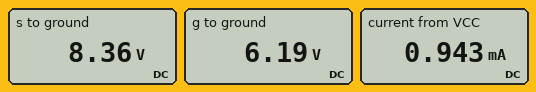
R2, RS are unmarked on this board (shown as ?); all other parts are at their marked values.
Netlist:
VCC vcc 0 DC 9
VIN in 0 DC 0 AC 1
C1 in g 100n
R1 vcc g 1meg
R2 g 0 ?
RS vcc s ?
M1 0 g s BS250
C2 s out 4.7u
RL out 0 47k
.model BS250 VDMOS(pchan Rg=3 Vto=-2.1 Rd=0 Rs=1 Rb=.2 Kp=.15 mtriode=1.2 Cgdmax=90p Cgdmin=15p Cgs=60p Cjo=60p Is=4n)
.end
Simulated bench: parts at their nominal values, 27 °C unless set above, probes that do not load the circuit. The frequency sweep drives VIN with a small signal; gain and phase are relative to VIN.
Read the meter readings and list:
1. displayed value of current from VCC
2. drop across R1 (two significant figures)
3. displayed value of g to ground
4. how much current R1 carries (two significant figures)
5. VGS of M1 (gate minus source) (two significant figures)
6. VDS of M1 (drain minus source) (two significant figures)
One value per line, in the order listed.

0.943 mA
2.8 V
6.19 V
2.8 µA
-2.2 V
-8.4 V
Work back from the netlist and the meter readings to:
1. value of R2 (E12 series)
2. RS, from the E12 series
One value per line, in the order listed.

2.2 MΩ
680 Ω
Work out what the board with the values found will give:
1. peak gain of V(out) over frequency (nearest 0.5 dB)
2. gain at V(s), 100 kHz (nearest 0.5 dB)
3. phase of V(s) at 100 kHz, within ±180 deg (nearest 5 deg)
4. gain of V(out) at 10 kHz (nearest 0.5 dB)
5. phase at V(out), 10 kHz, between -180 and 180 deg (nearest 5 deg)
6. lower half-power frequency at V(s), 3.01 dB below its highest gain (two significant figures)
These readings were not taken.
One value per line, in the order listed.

-1.0 dB
-1.0 dB
0 deg
-1.0 dB
0 deg
2.3 Hz
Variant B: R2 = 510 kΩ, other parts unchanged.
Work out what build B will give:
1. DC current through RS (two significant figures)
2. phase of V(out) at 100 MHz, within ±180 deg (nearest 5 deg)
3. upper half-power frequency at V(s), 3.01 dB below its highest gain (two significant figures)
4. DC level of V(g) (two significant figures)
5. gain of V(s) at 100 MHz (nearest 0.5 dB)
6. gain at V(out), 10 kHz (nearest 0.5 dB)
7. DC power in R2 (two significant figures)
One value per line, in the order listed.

5.3 mA
-10 deg
580 MHz
3.0 V
-1.5 dB
-0.5 dB
18 µW
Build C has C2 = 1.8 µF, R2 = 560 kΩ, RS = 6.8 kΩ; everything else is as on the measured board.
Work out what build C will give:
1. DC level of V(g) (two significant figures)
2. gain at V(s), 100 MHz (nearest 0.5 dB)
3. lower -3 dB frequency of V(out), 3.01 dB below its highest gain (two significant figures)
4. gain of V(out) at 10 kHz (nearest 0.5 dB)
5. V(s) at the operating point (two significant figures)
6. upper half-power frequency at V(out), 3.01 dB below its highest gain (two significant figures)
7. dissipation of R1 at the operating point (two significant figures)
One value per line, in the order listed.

3.2 V
-2.5 dB
5.1 Hz
0 dB
5.4 V
460 MHz
33 µW
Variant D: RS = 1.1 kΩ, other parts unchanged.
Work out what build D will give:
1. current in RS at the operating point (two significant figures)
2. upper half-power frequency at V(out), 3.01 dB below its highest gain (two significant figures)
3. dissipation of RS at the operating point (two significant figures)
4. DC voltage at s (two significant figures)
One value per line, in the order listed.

610 µA
1.0 GHz
410 µW
8.3 V
